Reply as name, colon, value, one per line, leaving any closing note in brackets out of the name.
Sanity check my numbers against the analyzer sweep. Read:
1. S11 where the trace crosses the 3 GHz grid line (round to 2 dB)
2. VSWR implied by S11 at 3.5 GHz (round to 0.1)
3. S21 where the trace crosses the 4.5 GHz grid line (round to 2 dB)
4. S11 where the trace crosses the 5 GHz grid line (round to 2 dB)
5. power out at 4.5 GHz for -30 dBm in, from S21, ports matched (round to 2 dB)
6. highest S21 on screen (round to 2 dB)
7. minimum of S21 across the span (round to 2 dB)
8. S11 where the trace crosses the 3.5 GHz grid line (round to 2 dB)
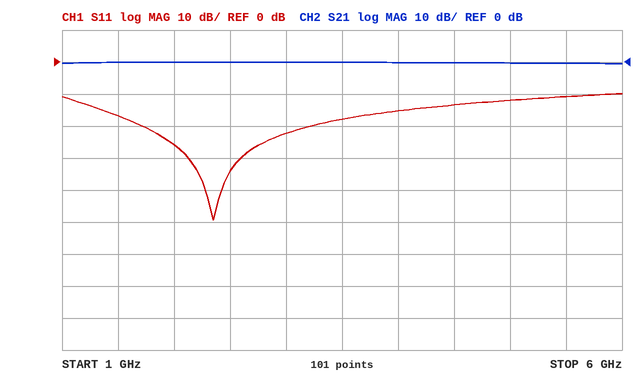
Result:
S11 where the trace crosses the 3 GHz grid line: -22 dB
VSWR implied by S11 at 3.5 GHz: 1.3
S21 where the trace crosses the 4.5 GHz grid line: 0 dB
S11 where the trace crosses the 5 GHz grid line: -12 dB
power out at 4.5 GHz for -30 dBm in, from S21, ports matched: -30 dBm
highest S21 on screen: 0 dB
minimum of S21 across the span: 0 dB
S11 where the trace crosses the 3.5 GHz grid line: -18 dB
